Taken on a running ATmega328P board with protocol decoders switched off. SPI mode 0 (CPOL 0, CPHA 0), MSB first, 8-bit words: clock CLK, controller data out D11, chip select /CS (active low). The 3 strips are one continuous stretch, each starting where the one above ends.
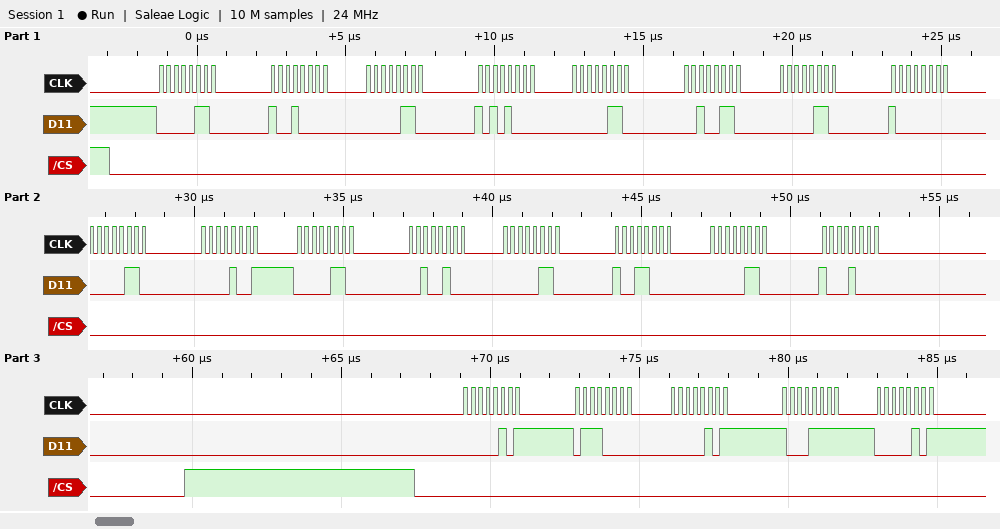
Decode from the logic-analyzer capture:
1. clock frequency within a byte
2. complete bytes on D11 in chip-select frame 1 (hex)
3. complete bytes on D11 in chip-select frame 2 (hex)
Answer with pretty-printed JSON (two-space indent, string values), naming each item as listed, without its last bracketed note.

{
  "clock frequency within a byte": "4 MHz",
  "complete bytes on D11 in chip-select frame 1": "0x06 0x90 0x06 0xA8 0x06 0x26 0x06 0x80 0x06 0x09 0x06 0x24 0x06 0x98 0x06 0x88",
  "complete bytes on D11 in chip-select frame 2": "0x05 0x70 0x05 0x8F 0x05"
}
